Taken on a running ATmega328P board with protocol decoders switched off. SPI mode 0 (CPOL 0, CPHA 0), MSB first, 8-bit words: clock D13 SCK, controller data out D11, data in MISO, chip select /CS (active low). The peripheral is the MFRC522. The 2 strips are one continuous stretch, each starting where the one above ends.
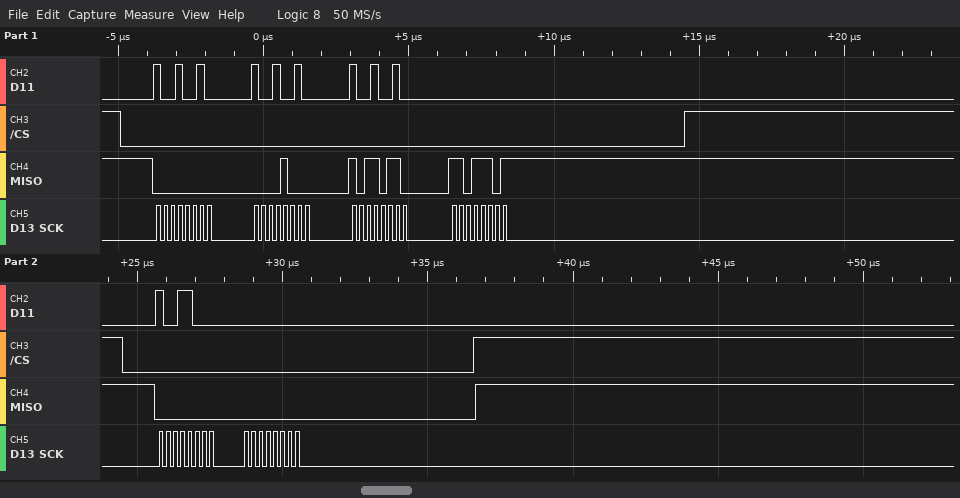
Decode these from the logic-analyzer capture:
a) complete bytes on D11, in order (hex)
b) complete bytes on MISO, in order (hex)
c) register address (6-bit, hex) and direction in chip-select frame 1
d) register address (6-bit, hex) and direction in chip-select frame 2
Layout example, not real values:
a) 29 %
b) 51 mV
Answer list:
a) 92 92 92 00 98 00
b) 00 08 B6 DD 00 00
c) 0x09 read
d) 0x0C read
